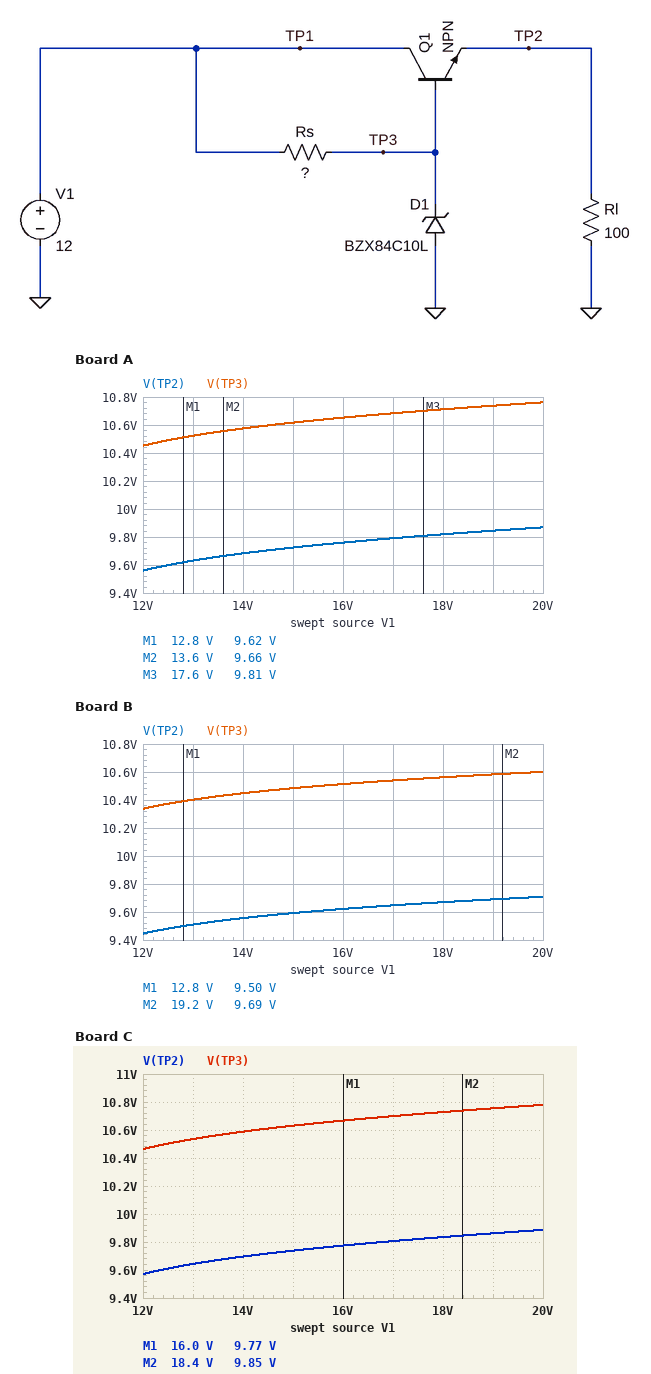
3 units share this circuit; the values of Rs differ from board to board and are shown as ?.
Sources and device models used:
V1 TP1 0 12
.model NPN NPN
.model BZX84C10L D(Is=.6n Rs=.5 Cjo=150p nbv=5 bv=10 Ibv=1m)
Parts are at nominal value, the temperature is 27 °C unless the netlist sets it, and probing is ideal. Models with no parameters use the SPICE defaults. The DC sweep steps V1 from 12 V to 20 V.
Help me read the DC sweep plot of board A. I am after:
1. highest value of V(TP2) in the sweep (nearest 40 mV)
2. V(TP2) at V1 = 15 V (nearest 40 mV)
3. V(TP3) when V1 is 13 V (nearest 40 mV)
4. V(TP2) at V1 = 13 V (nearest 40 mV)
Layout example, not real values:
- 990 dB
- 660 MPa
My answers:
- 9.88 V
- 9.72 V
- 10.52 V
- 9.64 V
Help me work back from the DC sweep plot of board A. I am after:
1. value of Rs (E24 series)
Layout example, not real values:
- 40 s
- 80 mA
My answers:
- 51 Ω
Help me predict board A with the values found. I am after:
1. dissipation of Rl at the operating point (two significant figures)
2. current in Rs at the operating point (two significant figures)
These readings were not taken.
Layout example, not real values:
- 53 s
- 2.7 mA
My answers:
- 910 mW
- 30 mA
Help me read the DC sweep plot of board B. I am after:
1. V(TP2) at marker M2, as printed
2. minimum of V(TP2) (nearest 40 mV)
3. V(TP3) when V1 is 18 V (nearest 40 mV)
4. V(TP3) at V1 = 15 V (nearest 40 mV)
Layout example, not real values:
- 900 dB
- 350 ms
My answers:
- 9.69 V
- 9.44 V
- 10.56 V
- 10.48 V
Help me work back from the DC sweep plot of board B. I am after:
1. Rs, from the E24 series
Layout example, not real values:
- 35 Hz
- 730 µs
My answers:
- 120 Ω
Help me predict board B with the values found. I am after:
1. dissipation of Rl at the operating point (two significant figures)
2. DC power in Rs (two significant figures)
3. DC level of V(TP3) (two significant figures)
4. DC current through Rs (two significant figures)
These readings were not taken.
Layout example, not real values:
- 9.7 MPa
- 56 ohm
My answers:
- 890 mW
- 23 mW
- 10 V
- 14 mA
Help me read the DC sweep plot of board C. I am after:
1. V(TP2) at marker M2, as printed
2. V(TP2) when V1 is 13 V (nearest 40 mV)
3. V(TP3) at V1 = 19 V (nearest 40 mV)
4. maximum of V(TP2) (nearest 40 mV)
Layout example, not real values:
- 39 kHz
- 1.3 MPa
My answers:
- 9.85 V
- 9.64 V
- 10.76 V
- 9.88 V
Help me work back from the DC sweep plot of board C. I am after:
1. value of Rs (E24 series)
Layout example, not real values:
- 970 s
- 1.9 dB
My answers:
- 47 Ω
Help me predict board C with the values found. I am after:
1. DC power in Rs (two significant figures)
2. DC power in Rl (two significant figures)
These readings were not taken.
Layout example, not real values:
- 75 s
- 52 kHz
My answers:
- 50 mW
- 920 mW
